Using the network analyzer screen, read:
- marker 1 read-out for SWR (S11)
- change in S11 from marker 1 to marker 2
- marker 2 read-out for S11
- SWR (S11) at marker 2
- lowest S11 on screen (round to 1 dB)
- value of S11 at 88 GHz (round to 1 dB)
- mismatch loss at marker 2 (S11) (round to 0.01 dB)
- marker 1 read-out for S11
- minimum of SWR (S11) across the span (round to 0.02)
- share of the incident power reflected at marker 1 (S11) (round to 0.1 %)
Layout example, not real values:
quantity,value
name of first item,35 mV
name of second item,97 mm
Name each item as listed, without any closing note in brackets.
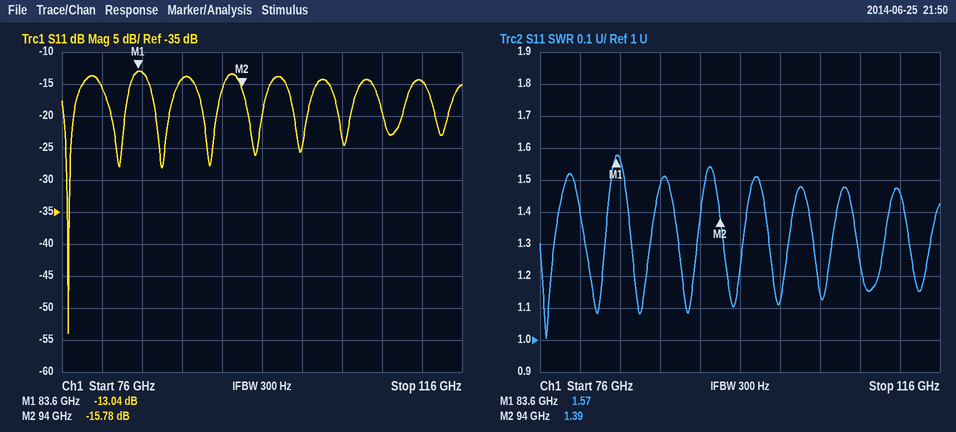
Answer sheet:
quantity,value
marker 1 read-out for SWR,1.57
change in S11 from marker 1 to marker 2,-2.74 dB
marker 2 read-out for S11,-15.78 dB
SWR (S11) at marker 2,1.39
lowest S11 on screen,-54 dB
value of S11 at 88 GHz,-14 dB
mismatch loss at marker 2 (S11),0.12 dB
marker 1 read-out for S11,-13.04 dB
minimum of SWR (S11) across the span,1.00
share of the incident power reflected at marker 1 (S11),5.0 %
